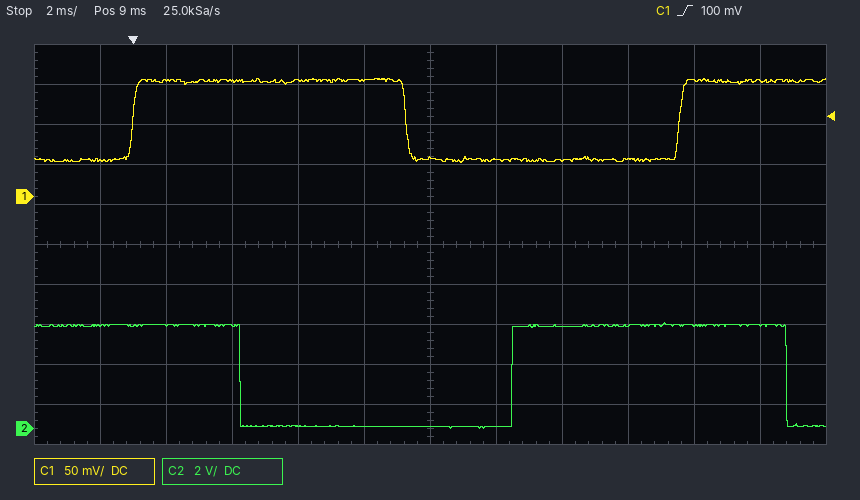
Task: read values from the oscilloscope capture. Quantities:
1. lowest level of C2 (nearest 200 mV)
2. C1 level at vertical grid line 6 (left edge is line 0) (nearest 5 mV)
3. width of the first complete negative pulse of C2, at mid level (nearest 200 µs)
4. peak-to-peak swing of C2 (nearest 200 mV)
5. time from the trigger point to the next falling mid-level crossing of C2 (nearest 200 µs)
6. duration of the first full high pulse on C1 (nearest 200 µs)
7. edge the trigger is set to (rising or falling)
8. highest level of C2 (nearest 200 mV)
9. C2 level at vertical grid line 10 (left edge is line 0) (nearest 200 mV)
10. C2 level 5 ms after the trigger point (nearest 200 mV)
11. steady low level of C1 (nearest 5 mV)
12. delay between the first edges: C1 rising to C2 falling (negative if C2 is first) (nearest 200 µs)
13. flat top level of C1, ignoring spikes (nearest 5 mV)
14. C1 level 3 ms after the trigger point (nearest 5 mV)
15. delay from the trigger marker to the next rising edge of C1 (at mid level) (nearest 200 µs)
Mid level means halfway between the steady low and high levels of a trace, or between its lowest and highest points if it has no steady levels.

0.0 V
50 mV
8.2 ms
5.2 V
3.2 ms
8.2 ms
rising
5.2 V
5.2 V
200 mV
45 mV
+3.2 ms
145 mV
145 mV
16.6 ms
